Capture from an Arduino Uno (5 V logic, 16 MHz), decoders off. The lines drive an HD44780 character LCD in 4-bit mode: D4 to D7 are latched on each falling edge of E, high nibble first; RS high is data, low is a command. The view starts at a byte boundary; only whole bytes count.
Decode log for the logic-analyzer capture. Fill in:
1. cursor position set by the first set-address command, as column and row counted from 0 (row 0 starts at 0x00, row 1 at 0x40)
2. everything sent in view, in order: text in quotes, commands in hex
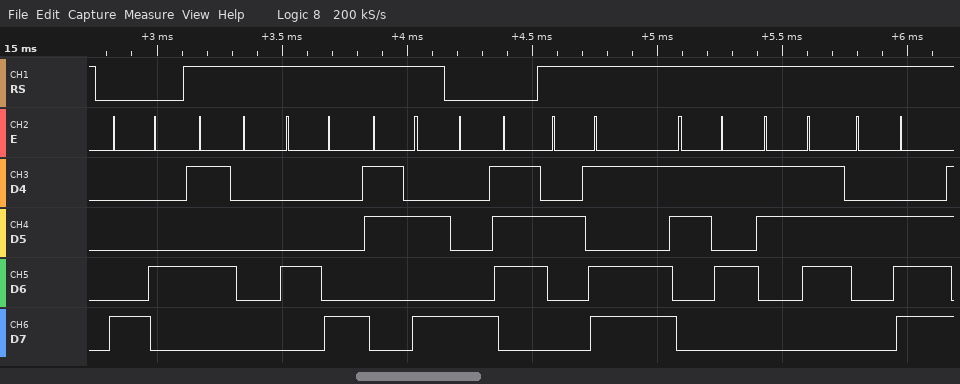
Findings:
column 4, row 0
0x84 "PH:" 0x87 "-57."
